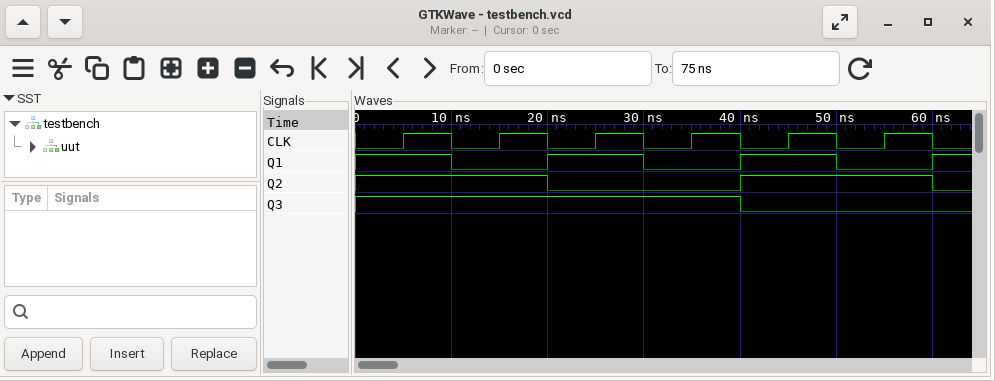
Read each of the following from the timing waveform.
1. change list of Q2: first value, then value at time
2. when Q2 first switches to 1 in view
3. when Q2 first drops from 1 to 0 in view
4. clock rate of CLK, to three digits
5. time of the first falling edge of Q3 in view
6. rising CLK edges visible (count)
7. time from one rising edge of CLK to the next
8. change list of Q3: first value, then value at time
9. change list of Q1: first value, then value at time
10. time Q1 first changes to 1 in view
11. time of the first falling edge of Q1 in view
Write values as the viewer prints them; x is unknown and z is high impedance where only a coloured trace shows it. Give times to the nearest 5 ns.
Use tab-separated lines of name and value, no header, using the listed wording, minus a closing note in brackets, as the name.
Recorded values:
change list of Q2: first value, then value at time	1, 0 at 20 ns, 1 at 40 ns, 0 at 60 ns
when Q2 first switches to 1 in view	40 ns
when Q2 first drops from 1 to 0 in view	20 ns
clock rate of CLK, to three digits	100 MHz
time of the first falling edge of Q3 in view	40 ns
rising CLK edges visible	6
time from one rising edge of CLK to the next	10 ns
change list of Q3: first value, then value at time	1, 0 at 40 ns
change list of Q1: first value, then value at time	1, 0 at 10 ns, 1 at 20 ns, 0 at 30 ns, 1 at 40 ns, 0 at 50 ns, 1 at 60 ns
time Q1 first changes to 1 in view	20 ns
time of the first falling edge of Q1 in view	10 ns
